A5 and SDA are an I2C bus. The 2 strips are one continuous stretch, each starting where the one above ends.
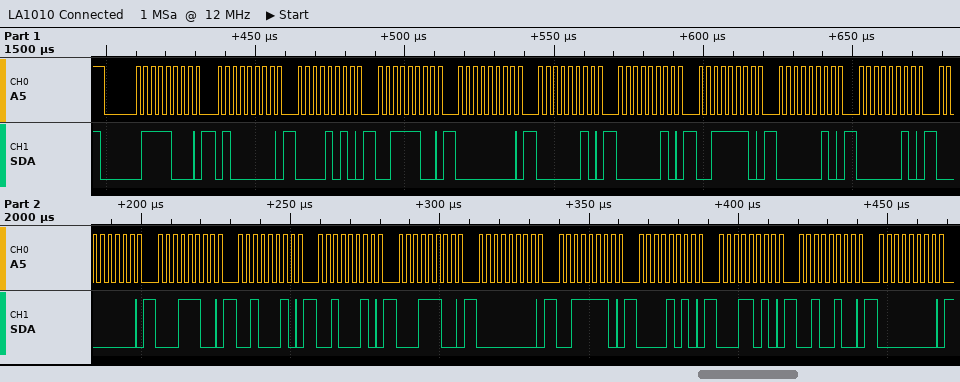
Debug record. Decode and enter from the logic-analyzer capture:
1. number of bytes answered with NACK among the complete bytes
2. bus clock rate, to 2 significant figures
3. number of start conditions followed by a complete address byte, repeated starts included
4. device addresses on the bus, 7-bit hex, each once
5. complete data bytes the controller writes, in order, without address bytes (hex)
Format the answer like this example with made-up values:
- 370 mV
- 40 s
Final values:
- 0
- 400 kHz
- 1
- 0x3C
- 40 0A 3C 00 02 02 3E 02 02 00 1C 22 22 1C 00 3E 0A 1A 24 00
